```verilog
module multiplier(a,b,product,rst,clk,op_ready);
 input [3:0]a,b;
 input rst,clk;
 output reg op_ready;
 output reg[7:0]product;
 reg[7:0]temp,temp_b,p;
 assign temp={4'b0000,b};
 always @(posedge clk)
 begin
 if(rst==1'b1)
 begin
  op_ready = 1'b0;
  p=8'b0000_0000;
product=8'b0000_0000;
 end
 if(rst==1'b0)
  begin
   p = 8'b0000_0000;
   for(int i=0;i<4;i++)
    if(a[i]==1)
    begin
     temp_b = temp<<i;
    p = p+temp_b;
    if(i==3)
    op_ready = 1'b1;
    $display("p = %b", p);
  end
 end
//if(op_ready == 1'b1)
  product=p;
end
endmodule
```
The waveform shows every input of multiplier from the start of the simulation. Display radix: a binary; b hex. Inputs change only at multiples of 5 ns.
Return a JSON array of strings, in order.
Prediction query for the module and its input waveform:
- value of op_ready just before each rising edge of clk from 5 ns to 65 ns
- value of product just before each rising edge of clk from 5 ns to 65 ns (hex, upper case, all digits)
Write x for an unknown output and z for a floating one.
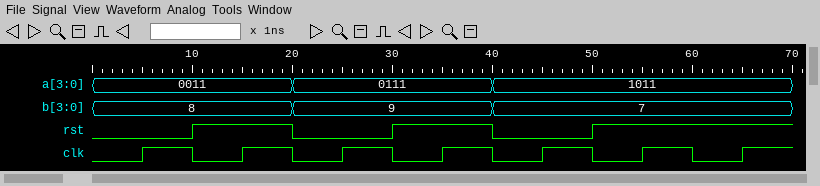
["x x 0 0 0 1 0", "x, 18, 00, 3F, 00, 4D, 00"]
